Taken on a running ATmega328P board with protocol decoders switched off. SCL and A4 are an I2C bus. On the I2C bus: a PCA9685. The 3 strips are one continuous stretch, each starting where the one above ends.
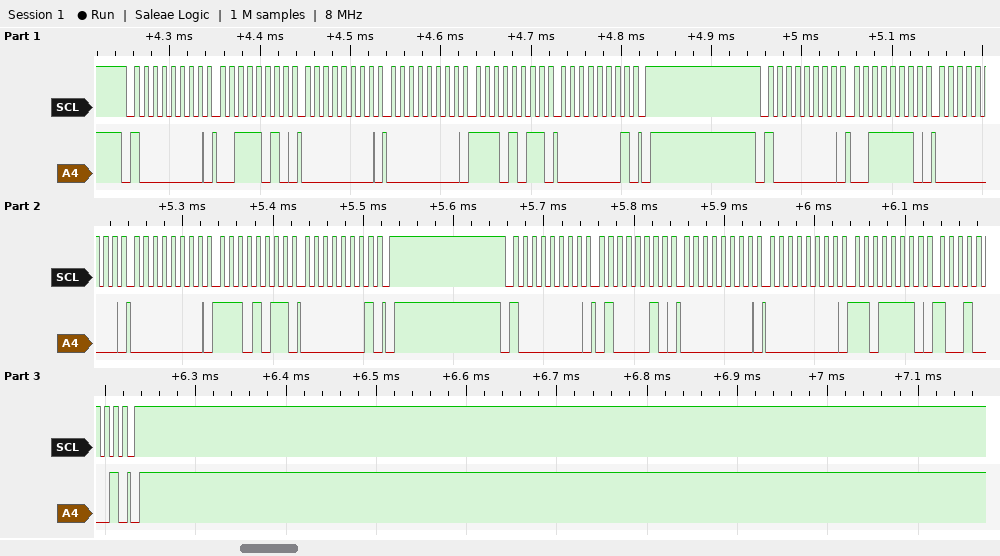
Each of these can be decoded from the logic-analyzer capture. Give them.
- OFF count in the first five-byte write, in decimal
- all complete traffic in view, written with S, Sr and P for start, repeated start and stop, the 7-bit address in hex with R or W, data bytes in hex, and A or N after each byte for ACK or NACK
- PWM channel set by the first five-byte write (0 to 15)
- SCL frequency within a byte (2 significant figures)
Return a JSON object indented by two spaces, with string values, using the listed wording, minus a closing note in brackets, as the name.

{
  "OFF count in the first five-byte write, in decimal": "491",
  "all complete traffic in view, written with S, Sr and P for start, repeated start and stop, the 7-bit address in hex with R or W, data bytes in hex, and A or N after each byte for ACK or NACK": "S 40W A 3A A 00 A 00 A EB A 01 A P S 40W A 3E A 00 A 00 A EB A 01 A P S 40W A 42 A 00 A 00 A DE A 91 A P",
  "PWM channel set by the first five-byte write": "13",
  "SCL frequency within a byte": "100 kHz"
}
